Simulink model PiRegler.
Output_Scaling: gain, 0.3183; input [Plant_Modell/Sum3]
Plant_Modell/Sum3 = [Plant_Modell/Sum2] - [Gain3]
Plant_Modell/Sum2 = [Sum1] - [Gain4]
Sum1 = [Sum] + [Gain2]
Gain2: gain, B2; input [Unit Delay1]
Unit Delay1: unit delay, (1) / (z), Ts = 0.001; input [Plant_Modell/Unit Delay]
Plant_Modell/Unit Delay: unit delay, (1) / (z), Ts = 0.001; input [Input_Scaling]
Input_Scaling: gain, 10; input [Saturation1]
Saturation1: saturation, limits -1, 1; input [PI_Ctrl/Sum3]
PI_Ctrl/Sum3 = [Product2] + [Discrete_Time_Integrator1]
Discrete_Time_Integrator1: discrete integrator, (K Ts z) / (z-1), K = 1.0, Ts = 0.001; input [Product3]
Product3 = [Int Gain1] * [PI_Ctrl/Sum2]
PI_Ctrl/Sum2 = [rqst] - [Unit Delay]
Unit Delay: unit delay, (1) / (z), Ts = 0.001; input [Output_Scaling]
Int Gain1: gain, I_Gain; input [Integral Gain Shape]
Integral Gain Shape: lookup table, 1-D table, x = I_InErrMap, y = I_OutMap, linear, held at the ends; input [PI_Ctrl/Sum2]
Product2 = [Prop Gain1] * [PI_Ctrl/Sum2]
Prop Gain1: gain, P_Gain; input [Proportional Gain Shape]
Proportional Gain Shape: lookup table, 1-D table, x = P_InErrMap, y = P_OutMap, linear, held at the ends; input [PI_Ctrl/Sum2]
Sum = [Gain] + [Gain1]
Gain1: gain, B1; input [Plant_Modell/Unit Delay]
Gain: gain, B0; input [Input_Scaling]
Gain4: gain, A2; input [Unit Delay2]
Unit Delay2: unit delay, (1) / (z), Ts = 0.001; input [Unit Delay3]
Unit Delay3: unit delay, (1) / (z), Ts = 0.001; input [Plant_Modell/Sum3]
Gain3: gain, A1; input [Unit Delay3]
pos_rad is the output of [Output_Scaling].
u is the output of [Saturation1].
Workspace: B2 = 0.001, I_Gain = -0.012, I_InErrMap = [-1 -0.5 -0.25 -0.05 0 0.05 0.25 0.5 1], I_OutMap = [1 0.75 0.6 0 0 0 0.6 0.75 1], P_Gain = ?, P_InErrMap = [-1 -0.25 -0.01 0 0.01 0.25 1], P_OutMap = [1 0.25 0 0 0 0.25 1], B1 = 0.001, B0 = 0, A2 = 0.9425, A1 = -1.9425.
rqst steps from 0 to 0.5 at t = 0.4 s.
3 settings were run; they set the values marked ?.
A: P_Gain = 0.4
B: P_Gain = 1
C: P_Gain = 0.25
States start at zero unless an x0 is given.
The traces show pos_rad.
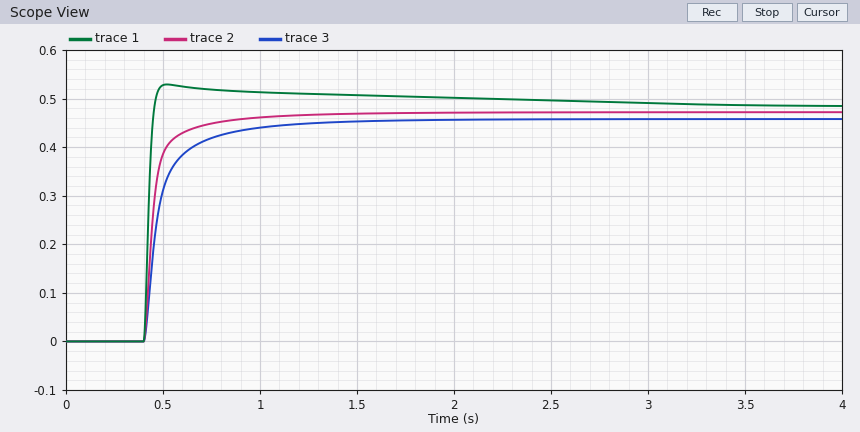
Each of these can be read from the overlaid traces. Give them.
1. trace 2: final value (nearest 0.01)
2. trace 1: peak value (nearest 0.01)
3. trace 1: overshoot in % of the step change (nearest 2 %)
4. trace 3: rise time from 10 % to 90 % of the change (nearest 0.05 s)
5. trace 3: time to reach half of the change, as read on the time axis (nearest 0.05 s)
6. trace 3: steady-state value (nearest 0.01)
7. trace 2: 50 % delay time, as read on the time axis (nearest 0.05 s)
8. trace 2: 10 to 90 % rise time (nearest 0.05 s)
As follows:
0.47
0.53
10 %
0.30 s
0.45 s
0.46
0.45 s
0.15 s
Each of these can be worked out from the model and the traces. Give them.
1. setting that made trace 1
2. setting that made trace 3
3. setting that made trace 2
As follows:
B
C
A
